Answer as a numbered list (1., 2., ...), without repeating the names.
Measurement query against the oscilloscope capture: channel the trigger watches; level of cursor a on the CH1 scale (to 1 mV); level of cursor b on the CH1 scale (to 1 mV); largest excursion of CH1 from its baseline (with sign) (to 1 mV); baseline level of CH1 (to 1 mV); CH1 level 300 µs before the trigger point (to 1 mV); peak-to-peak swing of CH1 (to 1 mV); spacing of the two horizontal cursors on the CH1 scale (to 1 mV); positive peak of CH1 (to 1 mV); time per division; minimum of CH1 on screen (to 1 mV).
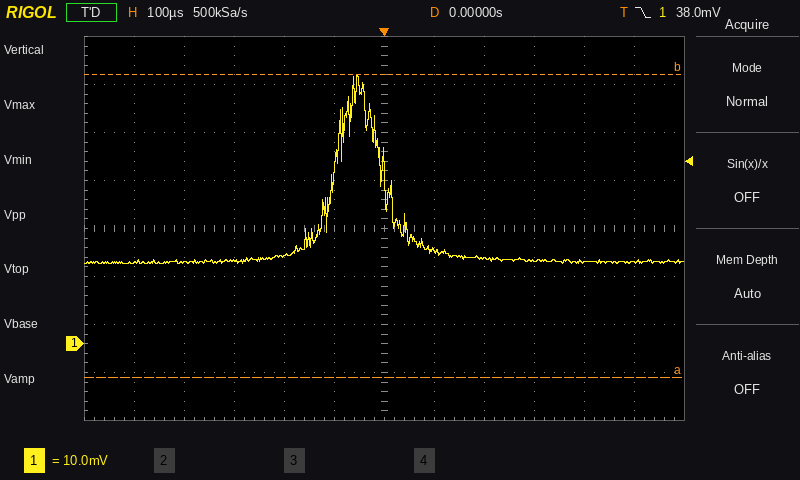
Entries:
1. CH1
2. -7 mV
3. 56 mV
4. +39 mV
5. 17 mV
6. 17 mV
7. 39 mV
8. 63 mV
9. 56 mV
10. 100 µs
11. 17 mV
